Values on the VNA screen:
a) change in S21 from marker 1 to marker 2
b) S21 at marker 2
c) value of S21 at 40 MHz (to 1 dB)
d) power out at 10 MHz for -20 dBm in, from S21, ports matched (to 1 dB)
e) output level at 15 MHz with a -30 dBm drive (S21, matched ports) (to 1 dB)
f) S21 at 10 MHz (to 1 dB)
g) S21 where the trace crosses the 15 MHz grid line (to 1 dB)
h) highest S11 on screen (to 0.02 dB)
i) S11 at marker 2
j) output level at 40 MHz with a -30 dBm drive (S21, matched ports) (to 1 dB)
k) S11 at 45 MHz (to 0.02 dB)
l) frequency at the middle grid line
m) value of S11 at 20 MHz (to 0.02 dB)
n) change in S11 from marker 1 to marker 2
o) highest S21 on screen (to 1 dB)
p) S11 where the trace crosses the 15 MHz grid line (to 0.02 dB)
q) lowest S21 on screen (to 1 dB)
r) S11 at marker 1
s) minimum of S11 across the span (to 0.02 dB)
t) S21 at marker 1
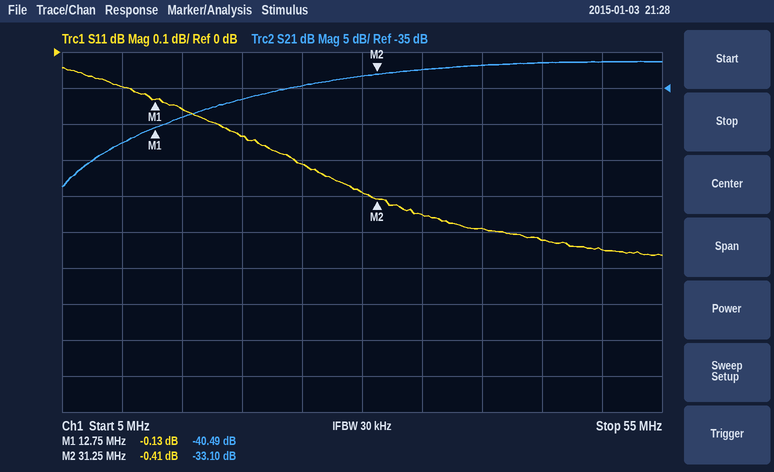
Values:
7.39 dB
-33.10 dB
-32 dB
-63 dBm
-69 dBm
-43 dB
-39 dB
-0.04 dB
-0.41 dB
-62 dBm
-0.52 dB
30 MHz
-0.24 dB
-0.28 dB
-31 dB
-0.16 dB
-49 dB
-0.13 dB
-0.56 dB
-40.49 dB
